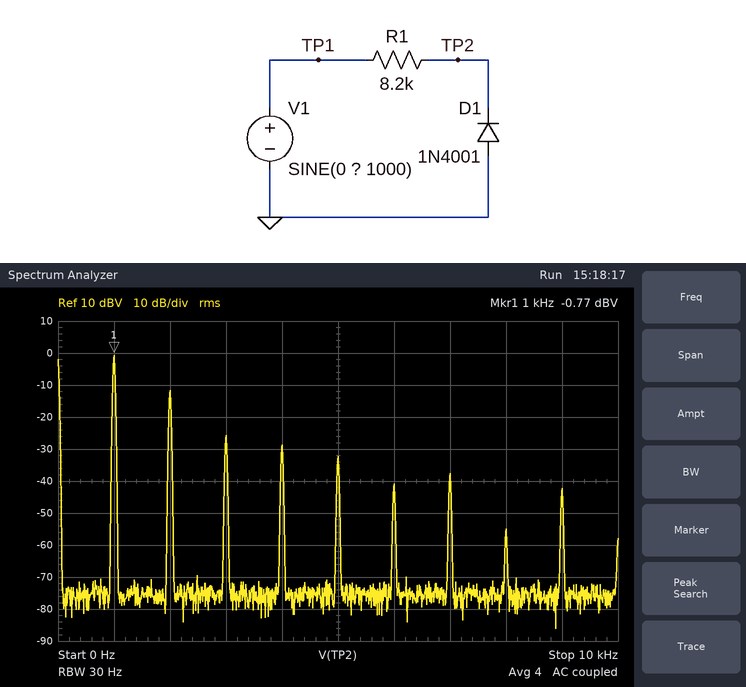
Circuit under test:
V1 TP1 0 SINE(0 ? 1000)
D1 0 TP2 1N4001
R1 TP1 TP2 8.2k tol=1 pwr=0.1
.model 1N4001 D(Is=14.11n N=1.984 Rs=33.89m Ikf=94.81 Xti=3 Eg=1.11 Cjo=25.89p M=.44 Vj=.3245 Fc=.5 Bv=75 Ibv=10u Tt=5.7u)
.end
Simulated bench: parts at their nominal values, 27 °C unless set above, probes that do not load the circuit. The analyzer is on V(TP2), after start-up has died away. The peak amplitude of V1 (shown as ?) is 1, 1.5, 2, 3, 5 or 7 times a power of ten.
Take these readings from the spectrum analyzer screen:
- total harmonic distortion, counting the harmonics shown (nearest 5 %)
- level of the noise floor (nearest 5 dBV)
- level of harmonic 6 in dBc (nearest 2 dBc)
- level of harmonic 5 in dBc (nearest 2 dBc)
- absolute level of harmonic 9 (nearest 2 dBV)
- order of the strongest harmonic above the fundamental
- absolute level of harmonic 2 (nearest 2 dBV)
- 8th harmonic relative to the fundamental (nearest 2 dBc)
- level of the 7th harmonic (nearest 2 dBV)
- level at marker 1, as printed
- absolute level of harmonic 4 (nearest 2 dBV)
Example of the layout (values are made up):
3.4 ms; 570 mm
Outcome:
30 %; -75 dBV; -40 dBc; -32 dBc; -42 dBV; 2; -12 dBV; -54 dBc; -38 dBV; -0.77 dBV; -28 dBV
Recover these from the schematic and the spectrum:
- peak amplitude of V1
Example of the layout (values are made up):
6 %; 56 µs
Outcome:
2 V
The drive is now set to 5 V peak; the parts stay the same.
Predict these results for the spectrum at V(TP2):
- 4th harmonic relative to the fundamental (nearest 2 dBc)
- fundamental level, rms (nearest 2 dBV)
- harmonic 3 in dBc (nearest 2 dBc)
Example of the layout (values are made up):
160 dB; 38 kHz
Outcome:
-24 dBc; 6 dBV; -30 dBc
